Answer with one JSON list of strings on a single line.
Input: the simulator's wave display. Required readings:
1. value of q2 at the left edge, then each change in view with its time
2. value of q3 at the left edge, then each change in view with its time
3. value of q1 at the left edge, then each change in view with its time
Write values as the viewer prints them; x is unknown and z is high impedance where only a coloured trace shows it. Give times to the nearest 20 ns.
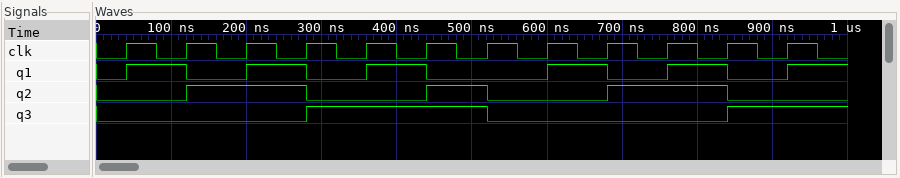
["0, 1 at 120 ns, 0 at 280 ns, 1 at 440 ns, 0 at 520 ns, 1 at 680 ns, 0 at 840 ns", "0, 1 at 280 ns, 0 at 520 ns, 1 at 840 ns", "0, 1 at 40 ns, 0 at 120 ns, 1 at 200 ns, 0 at 280 ns, 1 at 360 ns, 0 at 440 ns, 1 at 600 ns, 0 at 680 ns, 1 at 760 ns, 0 at 840 ns, 1 at 920 ns"]
